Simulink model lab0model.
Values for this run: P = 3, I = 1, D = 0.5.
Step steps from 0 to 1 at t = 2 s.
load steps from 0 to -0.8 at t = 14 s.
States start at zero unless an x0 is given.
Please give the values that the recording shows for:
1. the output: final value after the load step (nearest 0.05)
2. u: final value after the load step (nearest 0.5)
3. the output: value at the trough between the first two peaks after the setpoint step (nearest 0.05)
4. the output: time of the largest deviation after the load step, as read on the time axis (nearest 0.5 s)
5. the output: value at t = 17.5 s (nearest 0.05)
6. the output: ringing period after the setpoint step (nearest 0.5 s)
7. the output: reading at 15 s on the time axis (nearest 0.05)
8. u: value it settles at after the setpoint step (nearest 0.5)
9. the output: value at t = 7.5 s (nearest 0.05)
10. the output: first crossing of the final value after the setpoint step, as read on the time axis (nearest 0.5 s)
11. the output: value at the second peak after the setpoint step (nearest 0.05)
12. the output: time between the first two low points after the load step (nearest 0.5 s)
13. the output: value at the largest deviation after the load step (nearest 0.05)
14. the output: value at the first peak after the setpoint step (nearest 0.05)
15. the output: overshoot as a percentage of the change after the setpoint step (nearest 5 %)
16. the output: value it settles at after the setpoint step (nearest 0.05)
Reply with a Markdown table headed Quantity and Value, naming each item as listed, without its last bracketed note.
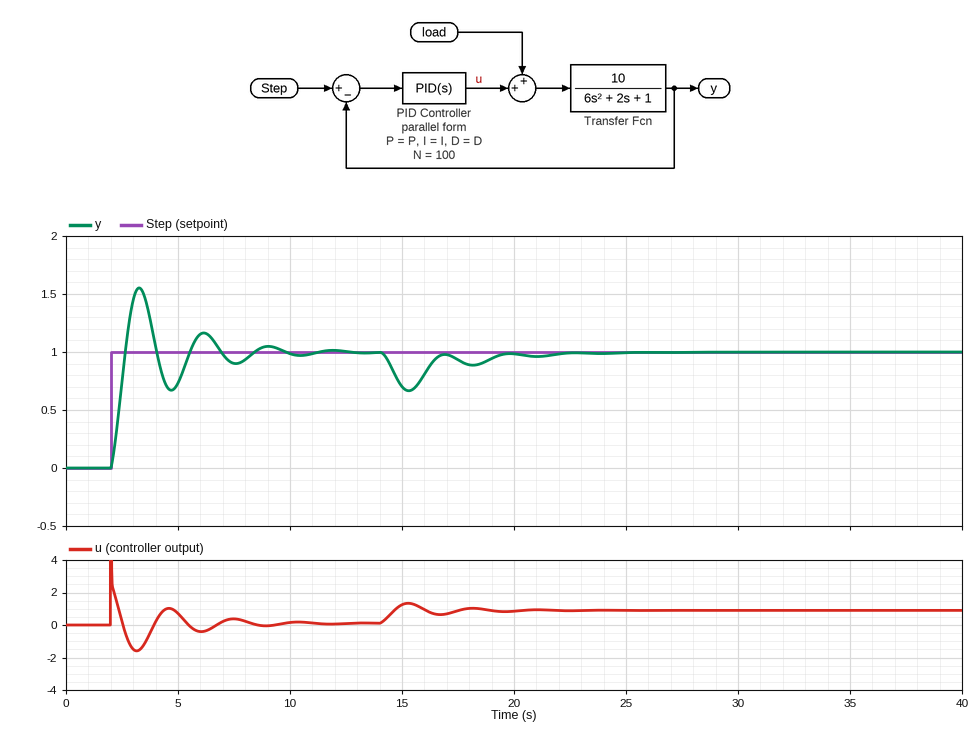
| Quantity | Value |
|---|---|
| the output: final value after the load step | 1.00 |
| u: final value after the load step | 1.0 |
| the output: value at the trough between the first two peaks after the setpoint step | 0.65 |
| the output: time of the largest deviation after the load step, as read on the time axis | 15.5 s |
| the output: value at t = 17.5 s | 0.95 |
| the output: ringing period after the setpoint step | 3.0 s |
| the output: reading at 15 s on the time axis | 0.70 |
| u: value it settles at after the setpoint step | 0.0 |
| the output: value at t = 7.5 s | 0.90 |
| the output: first crossing of the final value after the setpoint step, as read on the time axis | 2.5 s |
| the output: value at the second peak after the setpoint step | 1.15 |
| the output: time between the first two low points after the load step | 3.0 s |
| the output: value at the largest deviation after the load step | 0.65 |
| the output: value at the first peak after the setpoint step | 1.55 |
| the output: overshoot as a percentage of the change after the setpoint step | 55 % |
| the output: value it settles at after the setpoint step | 1.00 |
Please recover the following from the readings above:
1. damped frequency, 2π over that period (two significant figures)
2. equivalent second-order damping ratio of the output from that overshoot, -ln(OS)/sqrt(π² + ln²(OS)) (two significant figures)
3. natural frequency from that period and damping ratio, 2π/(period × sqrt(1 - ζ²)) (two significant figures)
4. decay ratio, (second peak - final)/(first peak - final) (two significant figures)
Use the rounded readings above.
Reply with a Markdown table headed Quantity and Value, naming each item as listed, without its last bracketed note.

| Quantity | Value |
|---|---|
| damped frequency, 2π over that period | 2.1 rad/s |
| equivalent second-order damping ratio of the output from that overshoot, -ln(OS)/sqrt(π² + ln²(OS)) | 0.19 |
| natural frequency from that period and damping ratio, 2π/(period × sqrt(1 - ζ²)) | 2.1 rad/s |
| decay ratio, (second peak - final)/(first peak - final) | 0.27 |
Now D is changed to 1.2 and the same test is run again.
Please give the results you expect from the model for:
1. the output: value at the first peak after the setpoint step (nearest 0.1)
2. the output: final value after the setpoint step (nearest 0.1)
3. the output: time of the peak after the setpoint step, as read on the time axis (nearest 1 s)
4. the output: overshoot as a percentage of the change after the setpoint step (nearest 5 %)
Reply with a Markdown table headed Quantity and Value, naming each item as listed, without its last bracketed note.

| Quantity | Value |
|---|---|
| the output: value at the first peak after the setpoint step | 1.3 |
| the output: final value after the setpoint step | 1.0 |
| the output: time of the peak after the setpoint step, as read on the time axis | 3 s |
| the output: overshoot as a percentage of the change after the setpoint step | 30 % |
